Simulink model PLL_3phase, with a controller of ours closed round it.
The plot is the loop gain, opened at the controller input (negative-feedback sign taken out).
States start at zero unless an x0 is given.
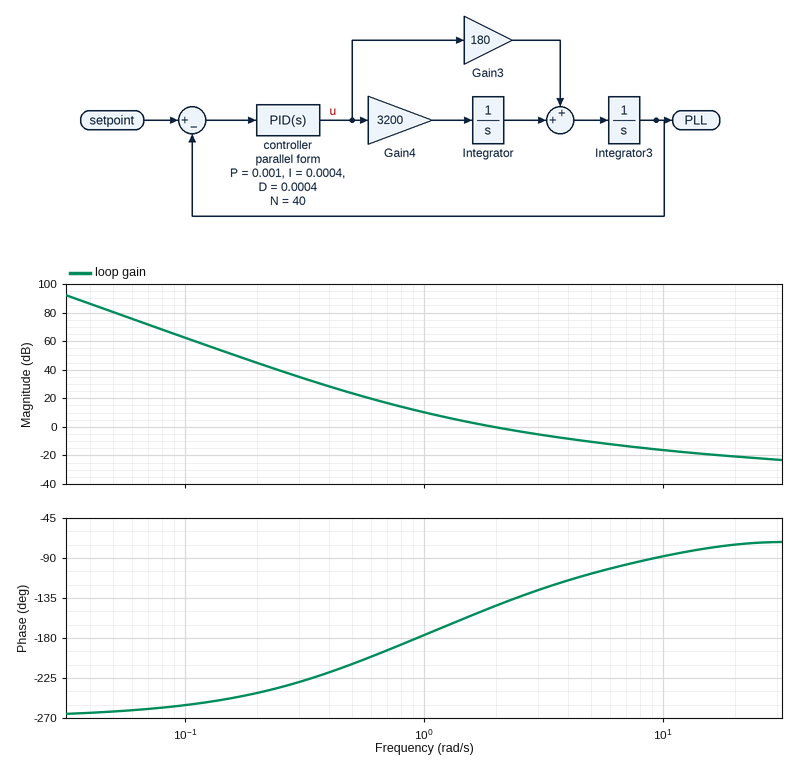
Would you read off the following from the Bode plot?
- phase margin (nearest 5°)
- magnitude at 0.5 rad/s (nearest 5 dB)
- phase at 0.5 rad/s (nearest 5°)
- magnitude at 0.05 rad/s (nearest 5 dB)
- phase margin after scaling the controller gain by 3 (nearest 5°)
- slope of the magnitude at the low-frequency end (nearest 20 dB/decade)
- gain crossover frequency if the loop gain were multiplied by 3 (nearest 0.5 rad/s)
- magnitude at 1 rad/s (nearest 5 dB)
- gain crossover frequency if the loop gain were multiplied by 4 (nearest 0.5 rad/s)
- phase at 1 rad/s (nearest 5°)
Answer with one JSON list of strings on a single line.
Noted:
["35°", "25 dB", "-210°", "80 dB", "70°", "-60 dB/decade", "4.5 rad/s", "10 dB", "6.0 rad/s", "-175°"]
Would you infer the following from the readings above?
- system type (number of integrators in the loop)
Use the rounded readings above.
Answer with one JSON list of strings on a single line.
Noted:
["3"]
